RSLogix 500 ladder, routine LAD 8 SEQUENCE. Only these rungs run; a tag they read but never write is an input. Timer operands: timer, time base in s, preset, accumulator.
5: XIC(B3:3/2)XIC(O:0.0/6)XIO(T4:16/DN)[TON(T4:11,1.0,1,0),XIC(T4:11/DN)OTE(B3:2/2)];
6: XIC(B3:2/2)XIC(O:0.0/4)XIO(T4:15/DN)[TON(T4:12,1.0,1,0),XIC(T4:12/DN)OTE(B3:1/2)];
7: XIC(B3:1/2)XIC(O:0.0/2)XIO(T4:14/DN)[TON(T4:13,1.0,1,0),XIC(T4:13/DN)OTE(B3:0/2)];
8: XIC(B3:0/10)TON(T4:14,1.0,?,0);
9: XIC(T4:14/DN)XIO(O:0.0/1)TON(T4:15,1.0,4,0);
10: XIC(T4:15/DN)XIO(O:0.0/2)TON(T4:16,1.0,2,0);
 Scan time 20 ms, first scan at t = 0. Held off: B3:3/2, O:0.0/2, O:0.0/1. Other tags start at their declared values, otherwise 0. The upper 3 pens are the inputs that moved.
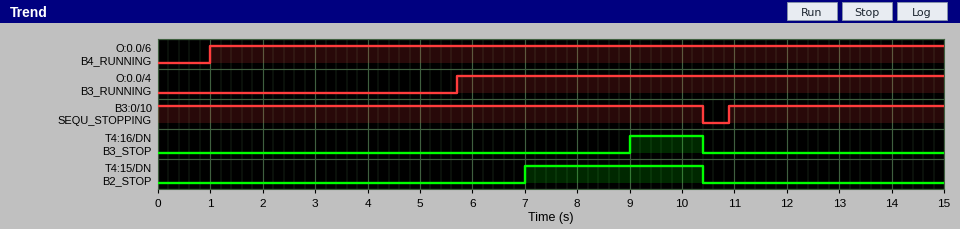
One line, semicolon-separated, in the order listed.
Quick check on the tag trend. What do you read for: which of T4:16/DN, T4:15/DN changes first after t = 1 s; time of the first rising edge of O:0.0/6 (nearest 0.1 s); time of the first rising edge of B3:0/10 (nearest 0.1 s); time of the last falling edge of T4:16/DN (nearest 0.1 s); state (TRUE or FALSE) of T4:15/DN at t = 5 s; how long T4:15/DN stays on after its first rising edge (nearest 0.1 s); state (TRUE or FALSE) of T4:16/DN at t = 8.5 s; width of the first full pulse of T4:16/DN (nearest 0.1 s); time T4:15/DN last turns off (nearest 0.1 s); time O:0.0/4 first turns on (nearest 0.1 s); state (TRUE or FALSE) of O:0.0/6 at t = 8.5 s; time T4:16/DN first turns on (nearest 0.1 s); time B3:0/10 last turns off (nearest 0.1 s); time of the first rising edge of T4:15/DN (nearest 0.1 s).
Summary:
T4:15/DN; 1.0 s; 10.9 s; 10.4 s; FALSE; 3.4 s; FALSE; 1.4 s; 10.4 s; 5.7 s; TRUE; 9.0 s; 10.4 s; 7.0 s
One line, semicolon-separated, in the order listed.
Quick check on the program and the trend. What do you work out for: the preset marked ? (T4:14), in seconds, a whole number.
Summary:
3 s
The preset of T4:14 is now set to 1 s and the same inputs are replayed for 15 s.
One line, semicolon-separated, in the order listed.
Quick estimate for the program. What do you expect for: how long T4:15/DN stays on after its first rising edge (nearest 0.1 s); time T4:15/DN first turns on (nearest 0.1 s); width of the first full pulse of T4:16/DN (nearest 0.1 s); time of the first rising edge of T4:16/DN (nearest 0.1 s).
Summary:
5.4 s; 5.0 s; 3.4 s; 7.0 s
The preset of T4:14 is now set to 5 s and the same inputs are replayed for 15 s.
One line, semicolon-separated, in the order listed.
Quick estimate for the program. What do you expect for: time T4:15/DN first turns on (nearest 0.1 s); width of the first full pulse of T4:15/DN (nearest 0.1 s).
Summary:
9.0 s; 1.4 s
